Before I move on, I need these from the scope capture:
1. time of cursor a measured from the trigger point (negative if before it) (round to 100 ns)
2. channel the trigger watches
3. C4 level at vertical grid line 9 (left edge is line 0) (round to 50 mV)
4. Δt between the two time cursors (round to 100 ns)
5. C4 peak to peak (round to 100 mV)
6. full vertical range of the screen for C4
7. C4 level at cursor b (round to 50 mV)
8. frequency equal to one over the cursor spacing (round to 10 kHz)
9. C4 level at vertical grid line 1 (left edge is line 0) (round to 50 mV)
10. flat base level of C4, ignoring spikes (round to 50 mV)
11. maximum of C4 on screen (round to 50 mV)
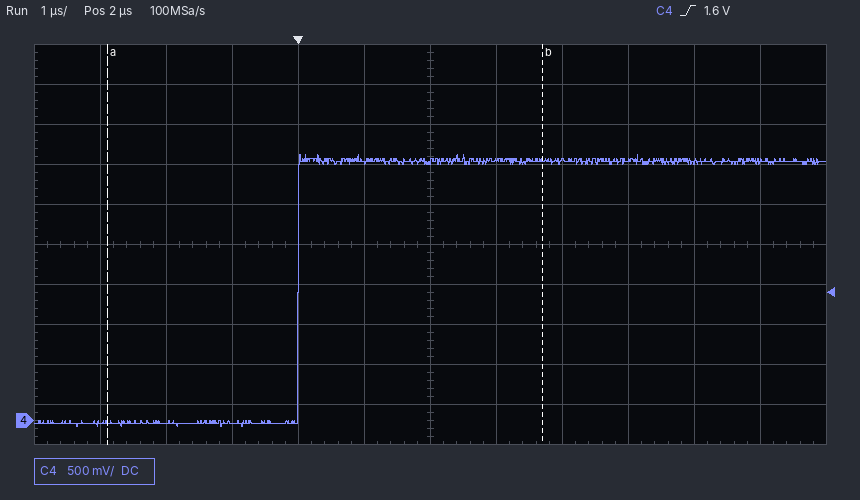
-2.9 µs
C4
3.25 V
6.6 µs
3.40 V
5 V
3.25 V
150 kHz
-50 mV
-50 mV
3.30 V
